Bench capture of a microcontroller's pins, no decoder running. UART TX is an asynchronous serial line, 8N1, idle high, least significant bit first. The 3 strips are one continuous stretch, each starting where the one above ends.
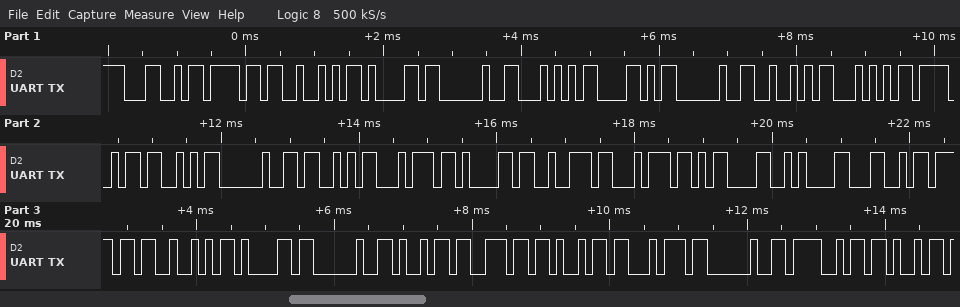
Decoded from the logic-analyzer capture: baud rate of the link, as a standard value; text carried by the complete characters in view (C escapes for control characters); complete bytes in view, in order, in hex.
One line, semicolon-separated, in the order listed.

9600 baud; "LoRa TX RTOS Start\r\nLoRa init OK"; 4C 6F 52 61 20 54 58 20 52 54 4F 53 20 53 74 61 72 74 0D 0A 4C 6F 52 61 20 69 6E 69 74 20 4F 4B
